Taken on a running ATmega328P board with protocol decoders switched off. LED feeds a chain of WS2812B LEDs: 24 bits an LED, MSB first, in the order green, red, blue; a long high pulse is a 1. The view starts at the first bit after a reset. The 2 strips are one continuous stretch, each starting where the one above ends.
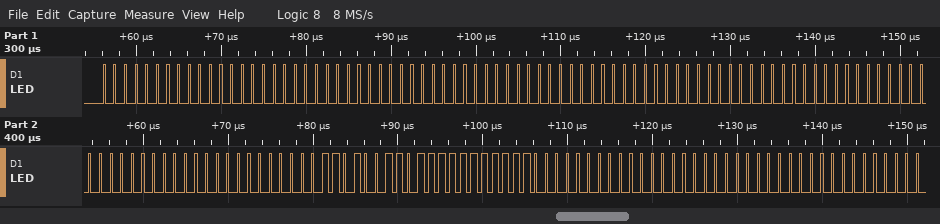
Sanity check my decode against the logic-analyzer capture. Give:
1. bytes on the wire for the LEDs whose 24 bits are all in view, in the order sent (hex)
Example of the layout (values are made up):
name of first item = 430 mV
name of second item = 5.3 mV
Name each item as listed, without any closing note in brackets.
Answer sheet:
bytes on the wire for the LEDs whose 24 bits are all in view, in the order sent = 00 00 00 00 00 00 00 00 00 00 00 00 0D 37 FF 00 00 00
